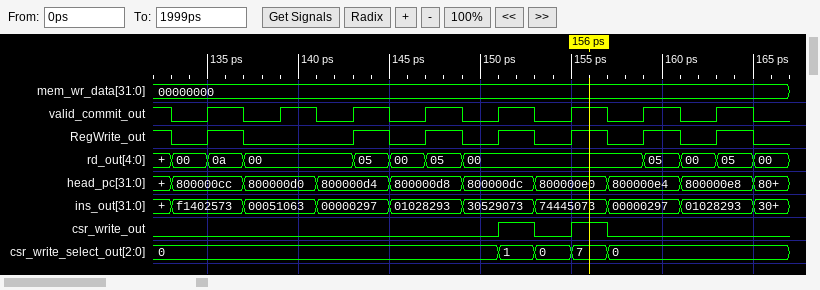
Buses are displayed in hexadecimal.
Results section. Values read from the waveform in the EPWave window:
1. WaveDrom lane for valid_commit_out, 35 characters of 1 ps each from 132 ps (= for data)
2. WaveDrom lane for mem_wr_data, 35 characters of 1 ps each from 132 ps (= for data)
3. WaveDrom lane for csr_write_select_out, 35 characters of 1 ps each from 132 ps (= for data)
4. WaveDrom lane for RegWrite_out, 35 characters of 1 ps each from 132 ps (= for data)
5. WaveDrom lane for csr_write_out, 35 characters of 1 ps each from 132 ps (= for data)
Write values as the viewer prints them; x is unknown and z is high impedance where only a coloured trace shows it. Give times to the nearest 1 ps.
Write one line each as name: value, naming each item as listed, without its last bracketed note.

WaveDrom lane for valid_commit_out, 35 characters of 1 ps each from 132 ps: {name: 'valid_commit_out', wave: '10.1.0.1.0.1.0.1.0.1.0.1.0.1.0.1.0.'}
WaveDrom lane for mem_wr_data, 35 characters of 1 ps each from 132 ps: {name: 'mem_wr_data', wave: '=..................................', data: '00000000'}
WaveDrom lane for csr_write_select_out, 35 characters of 1 ps each from 132 ps: {name: 'csr_write_select_out', wave: '=..................=.=.=.=.........', data: '0 1 0 7 0'}
WaveDrom lane for RegWrite_out, 35 characters of 1 ps each from 132 ps: {name: 'RegWrite_out', wave: '10.1.0.....1.0.1.0.1.0.1.0.1.0.1.0.'}
WaveDrom lane for csr_write_out, 35 characters of 1 ps each from 132 ps: {name: 'csr_write_out', wave: '0..................1.0.1.0.........'}
